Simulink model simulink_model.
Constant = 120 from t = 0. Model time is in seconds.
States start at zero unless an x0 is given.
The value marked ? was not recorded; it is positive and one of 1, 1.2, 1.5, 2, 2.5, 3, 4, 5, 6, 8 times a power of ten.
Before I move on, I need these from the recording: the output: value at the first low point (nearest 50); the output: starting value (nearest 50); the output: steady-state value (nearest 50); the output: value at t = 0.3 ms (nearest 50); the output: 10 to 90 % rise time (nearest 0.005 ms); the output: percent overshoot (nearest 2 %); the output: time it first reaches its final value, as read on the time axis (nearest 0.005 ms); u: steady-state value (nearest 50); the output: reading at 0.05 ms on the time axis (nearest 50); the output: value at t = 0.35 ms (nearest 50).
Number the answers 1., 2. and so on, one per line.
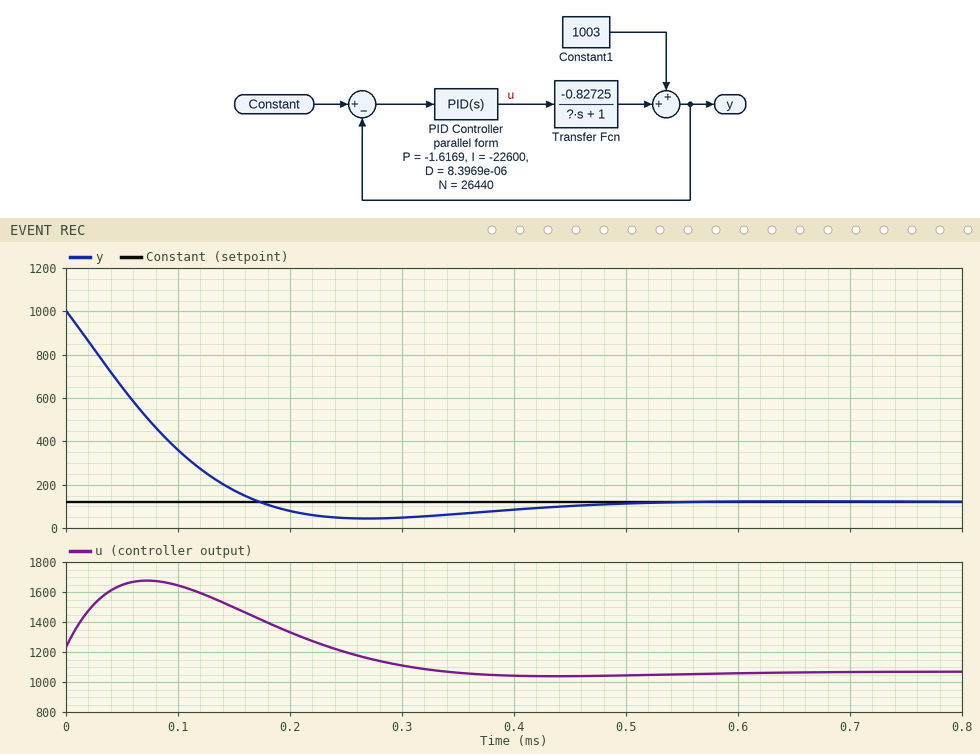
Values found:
1. 50
2. 1000
3. 100
4. 50
5. 0.125 ms
6. 8 %
7. 0.175 ms
8. 1050
9. 650
10. 50
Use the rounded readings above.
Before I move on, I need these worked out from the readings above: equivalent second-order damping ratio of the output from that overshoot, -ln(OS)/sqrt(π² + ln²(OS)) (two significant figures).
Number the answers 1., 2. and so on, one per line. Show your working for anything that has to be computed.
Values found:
1. ln(0.08) = -2.526; 2.526 / sqrt(9.870 + 6.379) = 0.63
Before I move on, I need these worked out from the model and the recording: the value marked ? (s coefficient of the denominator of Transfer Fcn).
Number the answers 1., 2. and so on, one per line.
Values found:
1. 0.00015
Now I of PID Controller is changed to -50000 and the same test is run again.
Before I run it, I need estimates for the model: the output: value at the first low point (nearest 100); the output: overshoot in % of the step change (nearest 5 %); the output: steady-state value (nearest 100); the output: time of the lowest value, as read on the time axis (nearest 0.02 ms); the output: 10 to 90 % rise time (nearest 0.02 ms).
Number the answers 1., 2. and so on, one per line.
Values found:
1. -100
2. 25 %
3. 100
4. 0.18 ms
5. 0.08 ms
